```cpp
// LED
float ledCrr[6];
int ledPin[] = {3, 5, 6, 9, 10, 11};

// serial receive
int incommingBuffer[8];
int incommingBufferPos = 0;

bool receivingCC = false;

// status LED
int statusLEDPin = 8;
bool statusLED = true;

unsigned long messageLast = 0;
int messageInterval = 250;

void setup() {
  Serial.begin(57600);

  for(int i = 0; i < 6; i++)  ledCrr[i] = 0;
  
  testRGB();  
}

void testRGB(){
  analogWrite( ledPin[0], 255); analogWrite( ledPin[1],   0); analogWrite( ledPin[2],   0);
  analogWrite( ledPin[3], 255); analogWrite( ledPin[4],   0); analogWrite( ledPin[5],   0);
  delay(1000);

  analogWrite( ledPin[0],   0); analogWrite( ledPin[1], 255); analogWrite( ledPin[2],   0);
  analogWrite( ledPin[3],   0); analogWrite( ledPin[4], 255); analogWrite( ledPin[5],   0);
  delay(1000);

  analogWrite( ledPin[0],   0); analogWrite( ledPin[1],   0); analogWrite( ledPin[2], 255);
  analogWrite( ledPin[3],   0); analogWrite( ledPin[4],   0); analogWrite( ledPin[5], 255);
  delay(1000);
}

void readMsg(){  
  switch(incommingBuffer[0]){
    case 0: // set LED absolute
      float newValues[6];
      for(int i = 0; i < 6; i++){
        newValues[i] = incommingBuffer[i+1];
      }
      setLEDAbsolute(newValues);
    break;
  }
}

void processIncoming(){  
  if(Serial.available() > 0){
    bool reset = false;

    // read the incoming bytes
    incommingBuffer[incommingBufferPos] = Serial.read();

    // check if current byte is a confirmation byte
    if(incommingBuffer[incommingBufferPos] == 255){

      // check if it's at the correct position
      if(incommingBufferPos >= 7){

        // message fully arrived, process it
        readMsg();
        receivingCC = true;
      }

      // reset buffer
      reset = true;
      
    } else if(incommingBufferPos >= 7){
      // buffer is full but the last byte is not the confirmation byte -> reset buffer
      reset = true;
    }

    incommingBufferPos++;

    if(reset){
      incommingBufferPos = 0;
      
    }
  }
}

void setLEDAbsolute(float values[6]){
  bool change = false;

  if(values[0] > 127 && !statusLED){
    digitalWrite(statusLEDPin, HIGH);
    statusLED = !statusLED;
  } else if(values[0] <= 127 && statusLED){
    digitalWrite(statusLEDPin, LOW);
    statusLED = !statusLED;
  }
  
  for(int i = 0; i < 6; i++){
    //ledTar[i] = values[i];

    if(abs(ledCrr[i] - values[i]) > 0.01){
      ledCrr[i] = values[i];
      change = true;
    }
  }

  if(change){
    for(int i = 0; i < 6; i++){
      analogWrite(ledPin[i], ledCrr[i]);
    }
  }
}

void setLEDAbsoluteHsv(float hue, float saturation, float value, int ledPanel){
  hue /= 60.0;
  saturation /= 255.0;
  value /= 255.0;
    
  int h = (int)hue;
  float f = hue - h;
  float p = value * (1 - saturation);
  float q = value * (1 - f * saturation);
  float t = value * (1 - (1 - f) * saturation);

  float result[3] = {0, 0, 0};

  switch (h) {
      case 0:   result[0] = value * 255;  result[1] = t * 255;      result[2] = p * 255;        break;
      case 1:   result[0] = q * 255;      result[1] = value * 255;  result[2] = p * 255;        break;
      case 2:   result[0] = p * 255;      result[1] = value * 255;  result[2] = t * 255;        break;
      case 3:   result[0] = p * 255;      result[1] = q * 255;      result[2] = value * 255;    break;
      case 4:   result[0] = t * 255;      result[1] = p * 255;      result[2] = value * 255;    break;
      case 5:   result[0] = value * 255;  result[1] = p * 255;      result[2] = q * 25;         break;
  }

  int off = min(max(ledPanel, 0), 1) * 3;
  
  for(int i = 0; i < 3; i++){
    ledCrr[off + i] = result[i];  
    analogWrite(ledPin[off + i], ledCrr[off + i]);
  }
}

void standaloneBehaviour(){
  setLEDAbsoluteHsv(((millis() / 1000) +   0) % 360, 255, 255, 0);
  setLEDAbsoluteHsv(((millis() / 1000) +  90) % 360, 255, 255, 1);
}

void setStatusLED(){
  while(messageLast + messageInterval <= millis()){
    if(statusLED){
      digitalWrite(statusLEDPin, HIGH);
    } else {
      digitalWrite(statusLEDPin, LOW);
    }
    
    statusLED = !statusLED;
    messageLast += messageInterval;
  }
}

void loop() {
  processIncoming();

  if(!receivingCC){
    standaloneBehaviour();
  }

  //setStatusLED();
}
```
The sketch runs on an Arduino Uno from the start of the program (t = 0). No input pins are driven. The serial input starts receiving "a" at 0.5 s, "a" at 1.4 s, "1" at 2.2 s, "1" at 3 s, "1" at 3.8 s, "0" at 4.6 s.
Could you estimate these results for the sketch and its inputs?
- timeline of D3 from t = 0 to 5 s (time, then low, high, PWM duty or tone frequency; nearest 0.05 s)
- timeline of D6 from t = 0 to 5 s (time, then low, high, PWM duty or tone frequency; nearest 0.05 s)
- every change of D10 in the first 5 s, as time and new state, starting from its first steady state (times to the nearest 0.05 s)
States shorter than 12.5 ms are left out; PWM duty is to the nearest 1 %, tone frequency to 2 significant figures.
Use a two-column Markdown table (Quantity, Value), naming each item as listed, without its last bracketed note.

| Quantity | Value |
|---|---|
| timeline of D3 from t = 0 to 5 s | 0 s high; 1 s low; 3 s high |
| timeline of D6 from t = 0 to 5 s | 0 s low; 2 s high; 3 s low |
| every change of D10 in the first 5 s, as time and new state, starting from its first steady state | 0 s low; 1 s high; 2 s low; 3 s high |
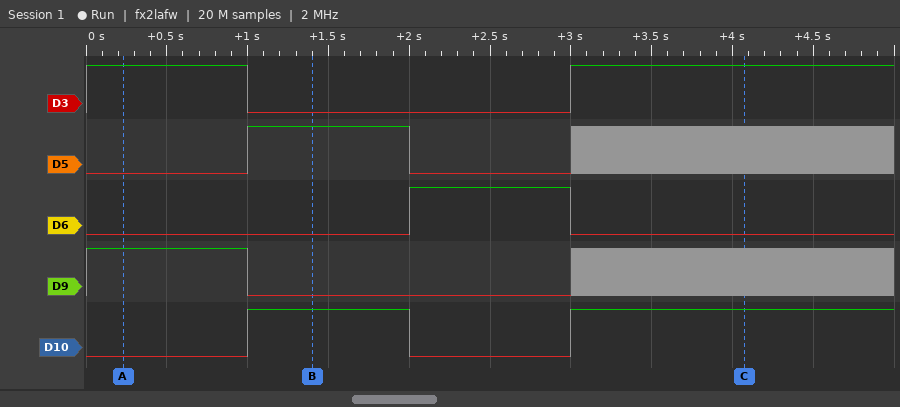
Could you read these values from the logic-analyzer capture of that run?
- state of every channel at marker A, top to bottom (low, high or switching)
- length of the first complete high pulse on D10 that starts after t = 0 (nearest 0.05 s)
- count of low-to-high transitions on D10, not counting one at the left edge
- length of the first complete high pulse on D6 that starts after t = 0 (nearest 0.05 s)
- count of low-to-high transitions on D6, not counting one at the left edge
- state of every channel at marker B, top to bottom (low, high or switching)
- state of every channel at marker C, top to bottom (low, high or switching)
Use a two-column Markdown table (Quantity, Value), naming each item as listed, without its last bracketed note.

| Quantity | Value |
|---|---|
| state of every channel at marker A, top to bottom | D3 high, D5 low, D6 low, D9 high, D10 low |
| length of the first complete high pulse on D10 that starts after t = 0 | 1.00 s |
| count of low-to-high transitions on D10, not counting one at the left edge | 2 |
| length of the first complete high pulse on D6 that starts after t = 0 | 1.00 s |
| count of low-to-high transitions on D6, not counting one at the left edge | 1 |
| state of every channel at marker B, top to bottom | D3 low, D5 high, D6 low, D9 low, D10 high |
| state of every channel at marker C, top to bottom | D3 high, D5 switching, D6 low, D9 switching, D10 high |
